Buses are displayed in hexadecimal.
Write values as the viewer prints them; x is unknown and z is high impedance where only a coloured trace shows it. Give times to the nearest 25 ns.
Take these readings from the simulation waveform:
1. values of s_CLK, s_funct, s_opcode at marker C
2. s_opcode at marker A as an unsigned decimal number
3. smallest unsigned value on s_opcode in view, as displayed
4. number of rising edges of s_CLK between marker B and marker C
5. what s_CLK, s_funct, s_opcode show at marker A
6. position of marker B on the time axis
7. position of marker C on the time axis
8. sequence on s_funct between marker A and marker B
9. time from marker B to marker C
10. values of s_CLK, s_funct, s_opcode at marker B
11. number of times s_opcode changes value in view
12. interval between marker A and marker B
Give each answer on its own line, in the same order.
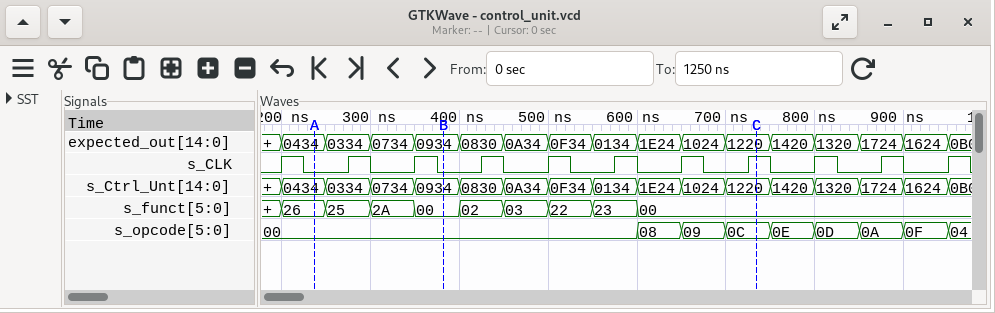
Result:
s_CLK=1, s_funct=00, s_opcode=0C
0
00
5
s_CLK=0, s_funct=26, s_opcode=00
375 ns
725 ns
26, 25, 2A, 00
350 ns
s_CLK=0, s_funct=00, s_opcode=00
8
150 ns
